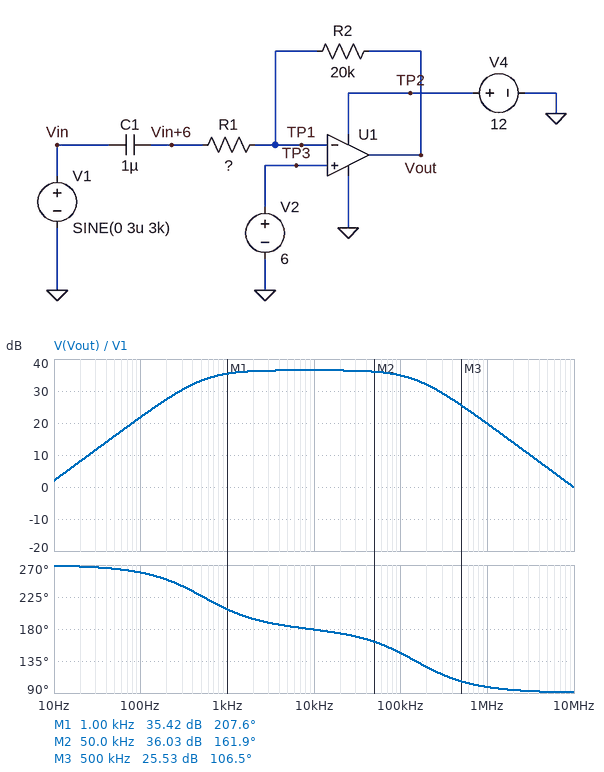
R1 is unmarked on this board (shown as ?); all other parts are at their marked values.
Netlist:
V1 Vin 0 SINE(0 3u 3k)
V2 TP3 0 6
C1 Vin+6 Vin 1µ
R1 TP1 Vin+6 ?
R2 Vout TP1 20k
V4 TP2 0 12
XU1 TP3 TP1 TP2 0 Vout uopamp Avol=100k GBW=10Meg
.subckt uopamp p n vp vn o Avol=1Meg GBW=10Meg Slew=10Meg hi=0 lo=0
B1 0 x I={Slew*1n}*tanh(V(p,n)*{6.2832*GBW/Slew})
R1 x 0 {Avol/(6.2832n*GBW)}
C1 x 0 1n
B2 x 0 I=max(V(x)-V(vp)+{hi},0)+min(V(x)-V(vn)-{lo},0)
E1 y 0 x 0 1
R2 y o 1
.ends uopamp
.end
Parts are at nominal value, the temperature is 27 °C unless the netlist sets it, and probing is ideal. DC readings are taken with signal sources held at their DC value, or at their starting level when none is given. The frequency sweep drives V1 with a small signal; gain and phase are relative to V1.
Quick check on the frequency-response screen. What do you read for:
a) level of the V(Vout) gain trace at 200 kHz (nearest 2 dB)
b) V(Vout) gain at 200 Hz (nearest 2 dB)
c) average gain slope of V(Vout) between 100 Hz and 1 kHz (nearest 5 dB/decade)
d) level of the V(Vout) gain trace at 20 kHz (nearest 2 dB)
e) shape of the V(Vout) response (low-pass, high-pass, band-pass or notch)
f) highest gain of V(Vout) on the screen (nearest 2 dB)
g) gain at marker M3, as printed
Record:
32 dB
28 dB
15 dB/decade
36 dB
band-pass
36 dB
25.53 dB
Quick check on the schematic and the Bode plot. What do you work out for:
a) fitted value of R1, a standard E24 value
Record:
300 Ω
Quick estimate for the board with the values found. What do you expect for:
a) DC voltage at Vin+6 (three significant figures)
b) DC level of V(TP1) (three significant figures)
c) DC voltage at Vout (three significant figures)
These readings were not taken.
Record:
6.00 V
6.00 V
6.00 V
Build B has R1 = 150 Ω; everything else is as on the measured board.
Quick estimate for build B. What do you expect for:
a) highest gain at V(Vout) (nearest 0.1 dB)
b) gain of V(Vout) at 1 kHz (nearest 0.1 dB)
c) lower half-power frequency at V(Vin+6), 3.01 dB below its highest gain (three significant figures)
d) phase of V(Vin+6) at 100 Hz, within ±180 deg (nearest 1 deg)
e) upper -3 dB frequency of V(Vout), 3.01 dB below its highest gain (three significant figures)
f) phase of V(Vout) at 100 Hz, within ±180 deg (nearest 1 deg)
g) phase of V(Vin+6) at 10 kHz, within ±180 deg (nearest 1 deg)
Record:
42.5 dB
39.3 dB
1.07 kHz
85 deg
75.6 kHz
-95 deg
6 deg
